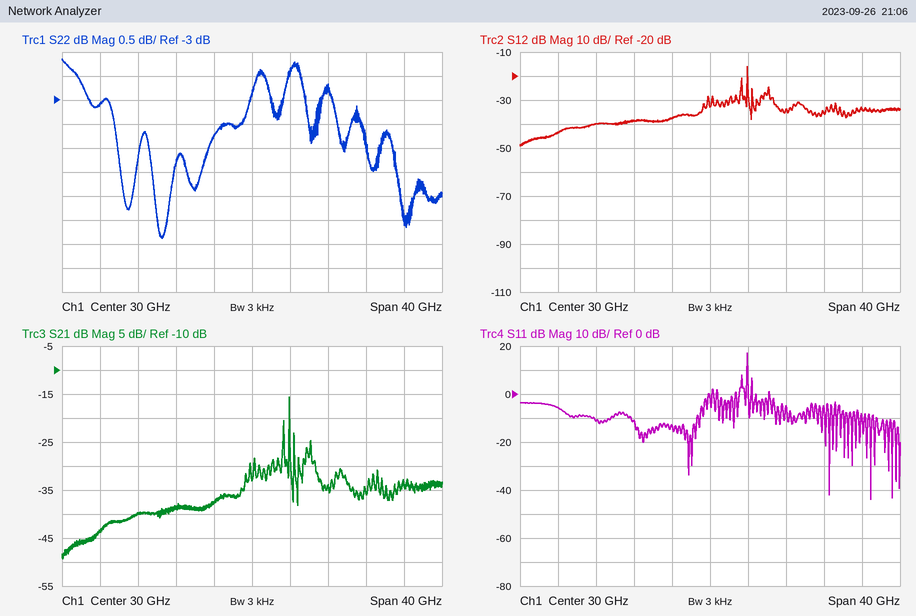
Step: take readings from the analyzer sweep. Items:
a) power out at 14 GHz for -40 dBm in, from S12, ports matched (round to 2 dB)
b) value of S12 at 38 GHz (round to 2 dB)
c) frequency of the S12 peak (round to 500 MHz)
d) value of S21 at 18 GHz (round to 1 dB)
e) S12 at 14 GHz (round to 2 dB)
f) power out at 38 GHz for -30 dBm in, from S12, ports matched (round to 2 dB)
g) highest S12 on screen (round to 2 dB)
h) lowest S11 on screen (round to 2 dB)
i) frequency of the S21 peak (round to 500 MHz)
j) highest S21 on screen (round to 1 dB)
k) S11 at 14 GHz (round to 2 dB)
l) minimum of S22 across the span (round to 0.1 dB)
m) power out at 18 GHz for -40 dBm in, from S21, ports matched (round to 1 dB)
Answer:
-84 dBm
-34 dB
34.0 GHz
-40 dB
-44 dB
-64 dBm
-16 dB
-44 dB
34.0 GHz
-16 dB
-6 dB
-5.9 dB
-80 dBm
